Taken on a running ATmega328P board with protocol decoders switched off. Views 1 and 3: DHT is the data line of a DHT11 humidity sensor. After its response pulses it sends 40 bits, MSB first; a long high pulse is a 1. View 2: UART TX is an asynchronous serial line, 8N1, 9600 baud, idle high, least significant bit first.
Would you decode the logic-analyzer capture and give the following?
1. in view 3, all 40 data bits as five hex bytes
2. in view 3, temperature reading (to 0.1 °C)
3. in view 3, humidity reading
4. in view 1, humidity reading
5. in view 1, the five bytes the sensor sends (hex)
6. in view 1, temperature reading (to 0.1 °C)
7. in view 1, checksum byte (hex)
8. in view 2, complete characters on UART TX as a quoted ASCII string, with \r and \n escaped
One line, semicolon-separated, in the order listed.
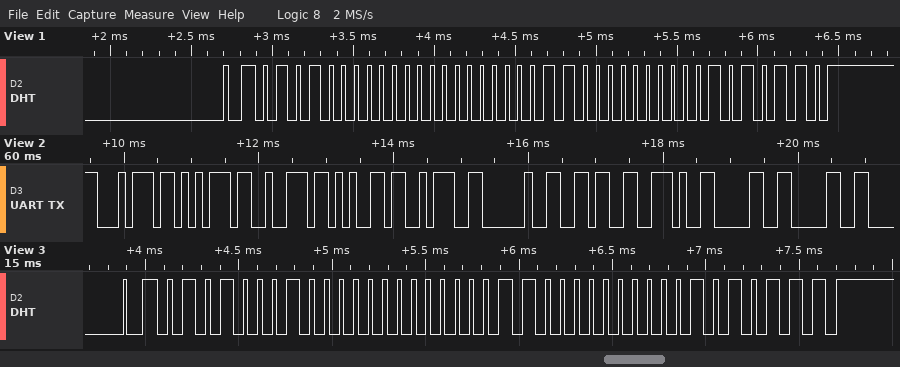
51 00 06 00 57; 6.0 °C; 81 %; 80 %; 50 00 06 00 56; 6.0 °C; 0x56; "ture: 6.00"
